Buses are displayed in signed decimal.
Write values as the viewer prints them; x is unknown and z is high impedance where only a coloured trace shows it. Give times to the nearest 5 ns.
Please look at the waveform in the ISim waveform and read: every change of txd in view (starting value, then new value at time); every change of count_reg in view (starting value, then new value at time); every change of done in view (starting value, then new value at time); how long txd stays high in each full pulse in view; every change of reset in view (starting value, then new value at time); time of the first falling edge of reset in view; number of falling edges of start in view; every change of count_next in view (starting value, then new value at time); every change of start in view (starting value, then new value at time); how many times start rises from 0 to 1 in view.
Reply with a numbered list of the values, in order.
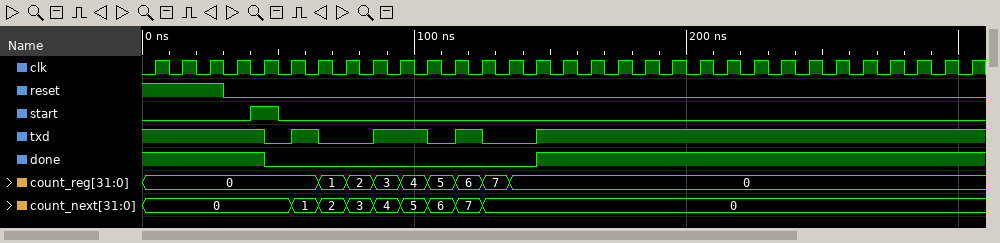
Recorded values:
1. 1, 0 at 45 ns, 1 at 55 ns, 0 at 65 ns, 1 at 85 ns, 0 at 105 ns, 1 at 115 ns, 0 at 125 ns, 1 at 145 ns
2. 0, 1 at 65 ns, 2 at 75 ns, 3 at 85 ns, 4 at 95 ns, 5 at 105 ns, 6 at 115 ns, 7 at 125 ns, 0 at 135 ns
3. 1, 0 at 45 ns, 1 at 145 ns
4. 10 ns, 20 ns, 10 ns
5. 1, 0 at 30 ns
6. 30 ns
7. 1
8. 0, 1 at 55 ns, 2 at 65 ns, 3 at 75 ns, 4 at 85 ns, 5 at 95 ns, 6 at 105 ns, 7 at 115 ns, 0 at 125 ns
9. 0, 1 at 40 ns, 0 at 50 ns
10. 1
